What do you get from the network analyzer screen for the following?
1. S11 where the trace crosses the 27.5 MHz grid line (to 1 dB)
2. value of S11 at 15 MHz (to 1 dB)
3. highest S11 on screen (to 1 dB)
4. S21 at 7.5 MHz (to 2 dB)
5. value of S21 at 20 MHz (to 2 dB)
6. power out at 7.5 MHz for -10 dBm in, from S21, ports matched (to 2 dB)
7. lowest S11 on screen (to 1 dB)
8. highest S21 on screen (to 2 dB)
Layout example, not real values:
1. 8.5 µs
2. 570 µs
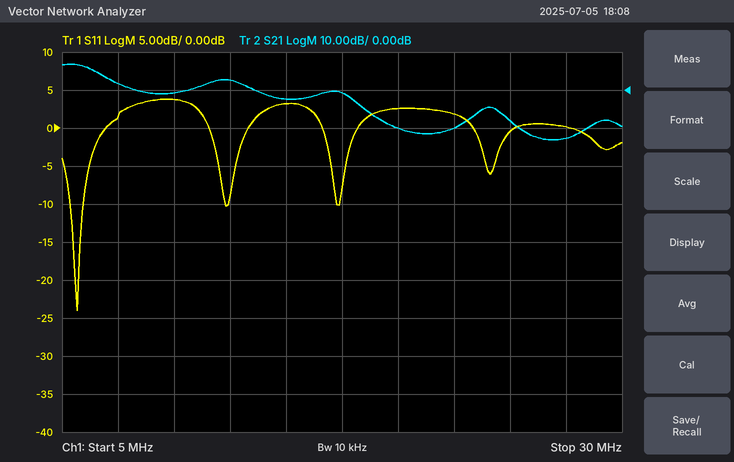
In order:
1. 0 dB
2. 3 dB
3. 4 dB
4. 2 dB
5. -10 dB
6. -8 dBm
7. -24 dB
8. 6 dB
